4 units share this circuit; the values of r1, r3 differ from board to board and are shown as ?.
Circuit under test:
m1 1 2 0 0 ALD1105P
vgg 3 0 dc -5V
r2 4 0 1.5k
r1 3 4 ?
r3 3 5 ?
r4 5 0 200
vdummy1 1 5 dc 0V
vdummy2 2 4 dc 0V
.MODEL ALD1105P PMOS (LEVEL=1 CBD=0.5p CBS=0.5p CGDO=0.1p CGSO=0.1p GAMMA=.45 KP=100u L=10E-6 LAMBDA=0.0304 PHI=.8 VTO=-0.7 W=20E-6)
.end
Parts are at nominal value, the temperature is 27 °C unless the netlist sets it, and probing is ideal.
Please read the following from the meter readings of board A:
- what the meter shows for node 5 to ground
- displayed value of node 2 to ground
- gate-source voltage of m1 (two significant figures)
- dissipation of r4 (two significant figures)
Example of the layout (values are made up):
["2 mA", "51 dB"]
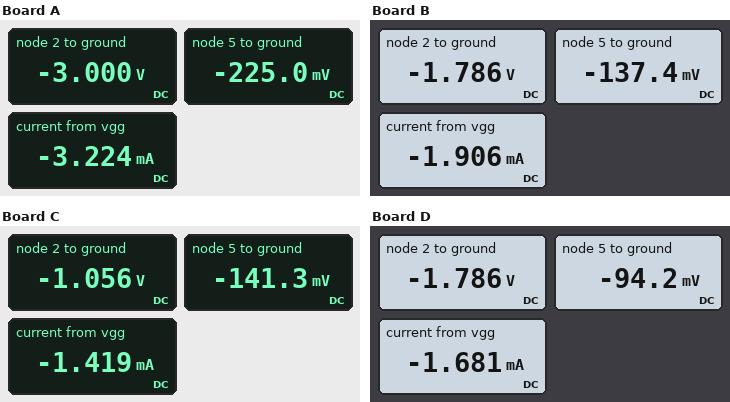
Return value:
["-225.0 mV", "-3.000 V", "-3.0 V", "250 µW"]
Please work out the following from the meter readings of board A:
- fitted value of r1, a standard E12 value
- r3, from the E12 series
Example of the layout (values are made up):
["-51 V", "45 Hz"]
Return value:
["1 kΩ", "3.9 kΩ"]
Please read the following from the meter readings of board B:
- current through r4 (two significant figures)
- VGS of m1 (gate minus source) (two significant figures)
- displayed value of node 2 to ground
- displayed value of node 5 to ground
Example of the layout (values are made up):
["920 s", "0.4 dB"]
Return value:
["690 µA", "-1.8 V", "-1.786 V", "-137.4 mV"]
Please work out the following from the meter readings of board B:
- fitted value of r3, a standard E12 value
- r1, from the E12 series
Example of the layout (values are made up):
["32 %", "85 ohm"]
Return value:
["6.8 kΩ", "2.7 kΩ"]
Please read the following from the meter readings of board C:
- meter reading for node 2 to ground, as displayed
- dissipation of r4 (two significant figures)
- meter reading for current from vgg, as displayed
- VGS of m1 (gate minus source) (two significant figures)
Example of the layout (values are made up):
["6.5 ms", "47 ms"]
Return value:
["-1.056 V", "100 µW", "-1.419 mA", "-1.1 V"]
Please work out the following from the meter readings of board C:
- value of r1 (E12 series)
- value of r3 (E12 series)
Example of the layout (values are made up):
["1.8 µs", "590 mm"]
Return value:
["5.6 kΩ", "6.8 kΩ"]
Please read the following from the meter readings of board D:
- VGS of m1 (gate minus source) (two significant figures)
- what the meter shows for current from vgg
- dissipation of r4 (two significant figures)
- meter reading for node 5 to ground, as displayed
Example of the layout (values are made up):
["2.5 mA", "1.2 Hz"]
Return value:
["-1.8 V", "-1.681 mA", "44 µW", "-94.2 mV"]
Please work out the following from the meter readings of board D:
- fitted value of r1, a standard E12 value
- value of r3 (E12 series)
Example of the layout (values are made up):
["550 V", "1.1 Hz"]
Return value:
["2.7 kΩ", "10 kΩ"]
